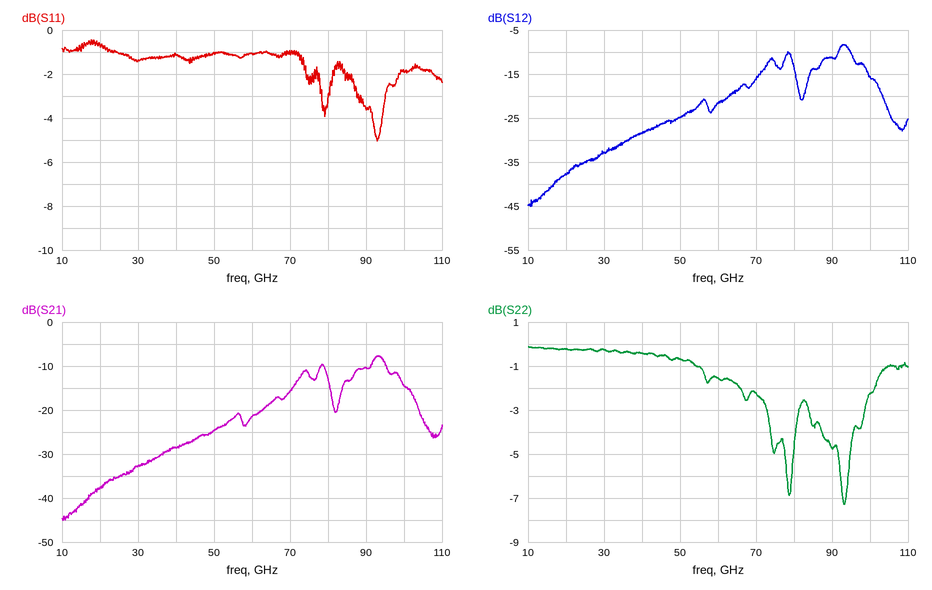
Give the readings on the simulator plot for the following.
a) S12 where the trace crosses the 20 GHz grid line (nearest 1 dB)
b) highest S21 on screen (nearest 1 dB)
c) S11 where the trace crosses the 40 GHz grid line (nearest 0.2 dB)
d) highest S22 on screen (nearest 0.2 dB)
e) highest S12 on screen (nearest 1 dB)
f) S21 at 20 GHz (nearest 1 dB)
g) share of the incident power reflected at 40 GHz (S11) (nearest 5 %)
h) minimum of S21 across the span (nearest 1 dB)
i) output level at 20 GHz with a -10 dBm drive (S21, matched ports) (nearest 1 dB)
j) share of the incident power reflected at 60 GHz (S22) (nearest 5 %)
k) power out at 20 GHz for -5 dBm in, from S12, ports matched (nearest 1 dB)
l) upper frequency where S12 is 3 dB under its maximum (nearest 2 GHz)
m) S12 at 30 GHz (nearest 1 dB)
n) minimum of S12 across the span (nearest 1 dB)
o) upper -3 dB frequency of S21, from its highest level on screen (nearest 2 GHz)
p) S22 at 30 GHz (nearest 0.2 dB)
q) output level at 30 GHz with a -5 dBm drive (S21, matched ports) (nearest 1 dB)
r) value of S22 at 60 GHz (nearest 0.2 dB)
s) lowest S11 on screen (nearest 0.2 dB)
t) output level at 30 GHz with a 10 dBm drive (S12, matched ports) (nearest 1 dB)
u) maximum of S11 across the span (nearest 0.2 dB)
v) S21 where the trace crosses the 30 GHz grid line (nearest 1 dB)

-38 dB
-8 dB
-1.2 dB
-0.2 dB
-8 dB
-38 dB
75 %
-45 dB
-48 dBm
70 %
-43 dBm
96 GHz
-33 dB
-45 dB
96 GHz
-0.2 dB
-38 dBm
-1.6 dB
-5.0 dB
-23 dBm
-0.4 dB
-33 dB
